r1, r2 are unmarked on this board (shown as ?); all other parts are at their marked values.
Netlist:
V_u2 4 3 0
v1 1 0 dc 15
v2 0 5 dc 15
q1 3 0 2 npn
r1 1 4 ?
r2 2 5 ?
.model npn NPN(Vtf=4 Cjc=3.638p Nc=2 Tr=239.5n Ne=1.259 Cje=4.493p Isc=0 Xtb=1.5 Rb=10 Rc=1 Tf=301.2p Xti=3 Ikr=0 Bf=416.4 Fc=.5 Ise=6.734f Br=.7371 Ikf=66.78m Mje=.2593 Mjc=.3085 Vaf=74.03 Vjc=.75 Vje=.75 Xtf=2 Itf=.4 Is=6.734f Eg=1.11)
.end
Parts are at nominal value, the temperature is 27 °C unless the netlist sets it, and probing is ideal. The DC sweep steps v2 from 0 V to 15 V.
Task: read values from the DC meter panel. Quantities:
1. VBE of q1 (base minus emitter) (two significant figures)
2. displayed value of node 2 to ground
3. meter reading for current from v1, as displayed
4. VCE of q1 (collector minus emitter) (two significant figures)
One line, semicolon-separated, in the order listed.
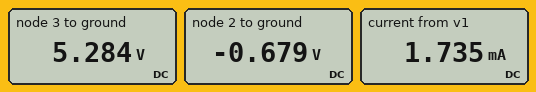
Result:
680 mV; -0.679 V; 1.735 mA; 6.0 V
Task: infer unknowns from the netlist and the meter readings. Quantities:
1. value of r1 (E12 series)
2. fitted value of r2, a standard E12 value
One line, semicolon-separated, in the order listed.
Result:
5.6 kΩ; 8.2 kΩ
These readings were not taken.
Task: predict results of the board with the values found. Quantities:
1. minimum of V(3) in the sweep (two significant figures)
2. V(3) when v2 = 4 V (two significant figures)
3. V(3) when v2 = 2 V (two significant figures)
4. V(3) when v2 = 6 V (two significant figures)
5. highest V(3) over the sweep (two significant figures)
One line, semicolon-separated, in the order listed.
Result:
5.3 V; 13 V; 14 V; 11 V; 15 V
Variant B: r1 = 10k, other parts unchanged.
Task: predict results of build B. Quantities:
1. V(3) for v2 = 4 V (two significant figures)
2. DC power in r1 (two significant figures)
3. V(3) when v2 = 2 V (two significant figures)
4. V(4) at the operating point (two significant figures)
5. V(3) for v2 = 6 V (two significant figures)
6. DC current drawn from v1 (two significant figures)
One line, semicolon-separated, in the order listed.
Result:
11 V; 24 mW; 13 V; -610 mV; 8.5 V; 1.6 mA
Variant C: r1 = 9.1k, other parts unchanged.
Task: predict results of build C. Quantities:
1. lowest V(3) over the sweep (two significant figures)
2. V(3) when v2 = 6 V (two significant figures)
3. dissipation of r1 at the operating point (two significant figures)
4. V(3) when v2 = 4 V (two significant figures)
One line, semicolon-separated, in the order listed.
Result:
-560 mV; 9.1 V; 27 mW; 11 V
